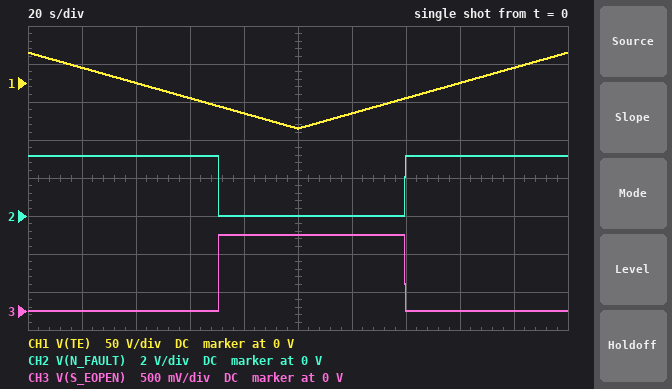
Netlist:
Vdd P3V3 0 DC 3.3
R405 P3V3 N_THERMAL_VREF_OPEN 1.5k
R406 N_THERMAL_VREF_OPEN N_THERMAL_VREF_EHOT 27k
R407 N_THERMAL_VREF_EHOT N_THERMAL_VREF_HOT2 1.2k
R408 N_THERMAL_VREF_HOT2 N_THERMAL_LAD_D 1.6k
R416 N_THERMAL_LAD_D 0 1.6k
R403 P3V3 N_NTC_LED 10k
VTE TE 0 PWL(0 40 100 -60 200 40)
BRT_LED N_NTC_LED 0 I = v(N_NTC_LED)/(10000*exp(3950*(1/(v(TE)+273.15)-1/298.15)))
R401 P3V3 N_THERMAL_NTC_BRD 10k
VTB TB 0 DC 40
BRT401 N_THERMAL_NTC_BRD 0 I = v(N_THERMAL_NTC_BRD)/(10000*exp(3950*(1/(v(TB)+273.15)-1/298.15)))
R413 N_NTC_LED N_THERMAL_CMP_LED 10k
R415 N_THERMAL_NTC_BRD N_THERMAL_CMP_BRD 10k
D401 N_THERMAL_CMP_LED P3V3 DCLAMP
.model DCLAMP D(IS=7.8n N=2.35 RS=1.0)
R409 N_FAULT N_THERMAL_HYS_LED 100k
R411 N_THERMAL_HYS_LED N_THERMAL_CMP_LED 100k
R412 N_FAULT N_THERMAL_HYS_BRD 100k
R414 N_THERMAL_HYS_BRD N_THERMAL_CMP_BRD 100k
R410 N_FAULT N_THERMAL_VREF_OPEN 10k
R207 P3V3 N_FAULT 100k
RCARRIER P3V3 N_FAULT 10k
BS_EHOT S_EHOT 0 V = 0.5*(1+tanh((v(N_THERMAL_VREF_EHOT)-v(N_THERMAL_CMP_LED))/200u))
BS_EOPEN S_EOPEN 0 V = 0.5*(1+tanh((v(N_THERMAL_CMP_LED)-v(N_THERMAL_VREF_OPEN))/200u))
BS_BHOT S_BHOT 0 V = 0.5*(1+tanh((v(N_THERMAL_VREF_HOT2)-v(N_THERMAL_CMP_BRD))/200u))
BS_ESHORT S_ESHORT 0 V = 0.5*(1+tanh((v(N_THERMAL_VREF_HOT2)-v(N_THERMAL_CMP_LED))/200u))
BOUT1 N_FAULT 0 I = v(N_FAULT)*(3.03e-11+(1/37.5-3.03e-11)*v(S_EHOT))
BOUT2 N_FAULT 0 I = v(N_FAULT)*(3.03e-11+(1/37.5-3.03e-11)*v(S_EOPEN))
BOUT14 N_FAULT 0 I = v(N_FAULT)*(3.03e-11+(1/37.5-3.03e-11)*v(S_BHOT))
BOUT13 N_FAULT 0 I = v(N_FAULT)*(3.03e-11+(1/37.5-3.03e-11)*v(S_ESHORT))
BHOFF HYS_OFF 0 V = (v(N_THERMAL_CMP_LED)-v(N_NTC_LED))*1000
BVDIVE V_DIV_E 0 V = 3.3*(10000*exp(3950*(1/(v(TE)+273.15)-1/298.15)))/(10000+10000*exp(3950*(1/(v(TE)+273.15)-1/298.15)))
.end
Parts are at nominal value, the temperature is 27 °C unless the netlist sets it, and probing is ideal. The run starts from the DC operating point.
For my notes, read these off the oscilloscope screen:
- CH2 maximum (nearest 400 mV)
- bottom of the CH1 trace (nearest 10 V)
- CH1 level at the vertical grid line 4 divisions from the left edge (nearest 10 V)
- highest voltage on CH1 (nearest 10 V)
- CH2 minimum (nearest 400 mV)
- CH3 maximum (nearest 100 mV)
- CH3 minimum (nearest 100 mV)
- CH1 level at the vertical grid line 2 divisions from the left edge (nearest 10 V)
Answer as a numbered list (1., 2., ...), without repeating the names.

1. 3.2 V
2. -60 V
3. -40 V
4. 40 V
5. 0 V
6. 1.0 V
7. 0 V
8. 0 V
